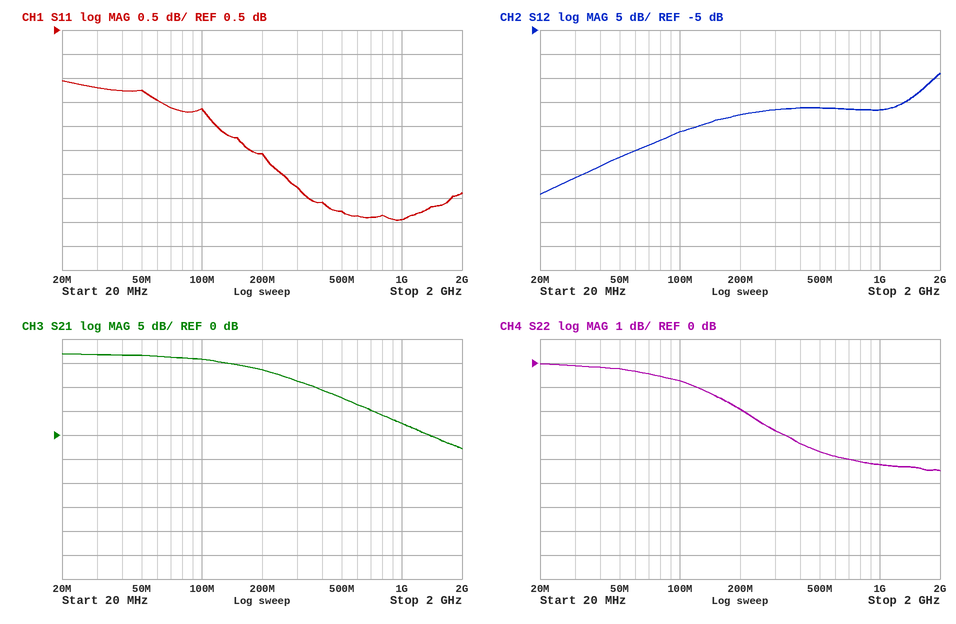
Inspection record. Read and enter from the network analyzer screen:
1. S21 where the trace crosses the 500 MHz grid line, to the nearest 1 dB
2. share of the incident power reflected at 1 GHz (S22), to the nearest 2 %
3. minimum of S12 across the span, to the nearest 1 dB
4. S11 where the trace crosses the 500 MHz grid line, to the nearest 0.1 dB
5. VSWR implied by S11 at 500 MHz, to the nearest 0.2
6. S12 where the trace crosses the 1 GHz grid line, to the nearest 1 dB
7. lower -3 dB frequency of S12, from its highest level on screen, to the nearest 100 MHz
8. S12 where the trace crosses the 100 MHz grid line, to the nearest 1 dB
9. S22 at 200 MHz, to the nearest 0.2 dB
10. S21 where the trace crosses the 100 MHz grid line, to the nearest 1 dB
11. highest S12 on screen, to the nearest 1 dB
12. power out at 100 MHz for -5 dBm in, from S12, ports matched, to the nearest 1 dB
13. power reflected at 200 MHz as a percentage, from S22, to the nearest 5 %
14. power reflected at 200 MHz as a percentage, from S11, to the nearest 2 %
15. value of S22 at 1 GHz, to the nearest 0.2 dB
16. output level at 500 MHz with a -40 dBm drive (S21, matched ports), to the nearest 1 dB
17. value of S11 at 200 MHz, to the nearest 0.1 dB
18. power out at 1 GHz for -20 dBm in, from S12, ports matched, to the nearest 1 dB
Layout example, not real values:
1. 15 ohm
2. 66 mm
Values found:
1. 8 dB
2. 38 %
3. -39 dB
4. -3.3 dB
5. 5.4
6. -22 dB
7. 1.7 GHz
8. -26 dB
9. -2.0 dB
10. 16 dB
11. -14 dB
12. -31 dBm
13. 65 %
14. 62 %
15. -4.2 dB
16. -32 dBm
17. -2.1 dB
18. -42 dBm
